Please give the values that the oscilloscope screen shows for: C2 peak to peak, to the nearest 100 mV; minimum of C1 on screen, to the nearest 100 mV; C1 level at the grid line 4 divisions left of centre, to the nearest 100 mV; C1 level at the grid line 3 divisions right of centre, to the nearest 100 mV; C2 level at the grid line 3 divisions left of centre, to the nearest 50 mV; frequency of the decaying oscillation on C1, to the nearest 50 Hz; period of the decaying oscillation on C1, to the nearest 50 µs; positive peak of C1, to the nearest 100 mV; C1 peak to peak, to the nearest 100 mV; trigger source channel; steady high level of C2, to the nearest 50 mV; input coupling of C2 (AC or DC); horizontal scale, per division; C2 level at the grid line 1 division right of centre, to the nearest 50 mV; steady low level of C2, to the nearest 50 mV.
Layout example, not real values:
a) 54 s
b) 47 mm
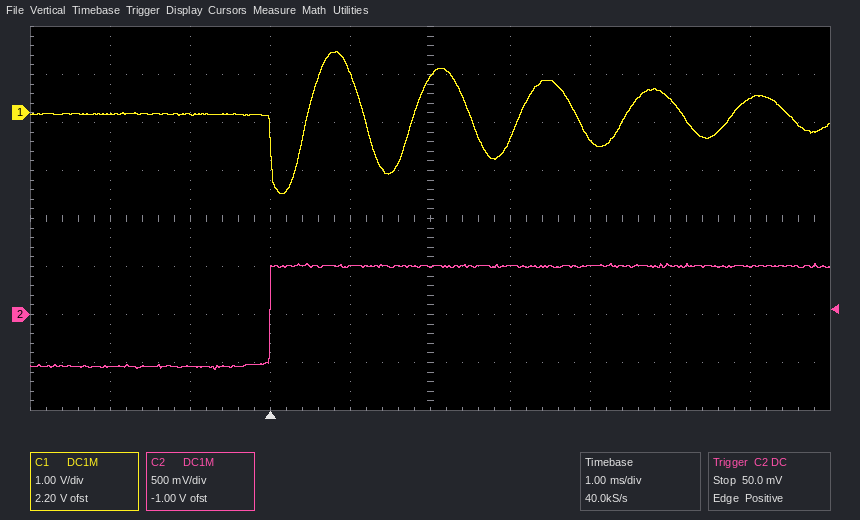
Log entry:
a) 1.10 V
b) -1.7 V
c) 0.0 V
d) 300 mV
e) -550 mV
f) 750 Hz
g) 1.30 ms
h) 1.3 V
i) 3.0 V
j) C2
k) 500 mV
l) DC
m) 1 ms
n) 500 mV
o) -550 mV
